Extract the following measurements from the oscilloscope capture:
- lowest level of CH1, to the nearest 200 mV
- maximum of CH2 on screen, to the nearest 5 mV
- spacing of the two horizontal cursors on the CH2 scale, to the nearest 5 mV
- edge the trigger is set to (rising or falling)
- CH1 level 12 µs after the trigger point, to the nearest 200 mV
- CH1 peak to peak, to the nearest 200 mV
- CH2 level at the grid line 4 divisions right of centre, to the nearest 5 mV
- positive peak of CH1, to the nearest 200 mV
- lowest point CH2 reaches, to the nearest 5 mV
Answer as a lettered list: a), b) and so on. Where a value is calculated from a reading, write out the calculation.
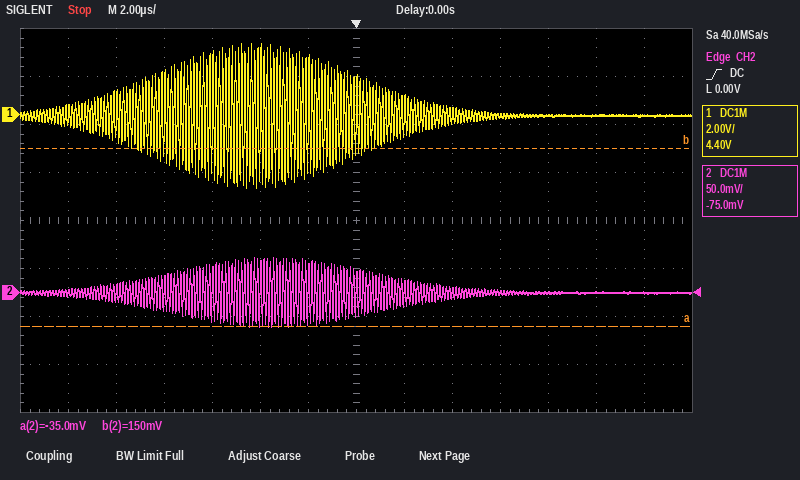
a) -3.0 V
b) 35 mV
c) 185 mV
d) rising
e) 0.0 V
f) 3.0 V − (-3.0 V) = 6.0 V
g) 0 mV
h) 3.0 V
i) -35 mV
